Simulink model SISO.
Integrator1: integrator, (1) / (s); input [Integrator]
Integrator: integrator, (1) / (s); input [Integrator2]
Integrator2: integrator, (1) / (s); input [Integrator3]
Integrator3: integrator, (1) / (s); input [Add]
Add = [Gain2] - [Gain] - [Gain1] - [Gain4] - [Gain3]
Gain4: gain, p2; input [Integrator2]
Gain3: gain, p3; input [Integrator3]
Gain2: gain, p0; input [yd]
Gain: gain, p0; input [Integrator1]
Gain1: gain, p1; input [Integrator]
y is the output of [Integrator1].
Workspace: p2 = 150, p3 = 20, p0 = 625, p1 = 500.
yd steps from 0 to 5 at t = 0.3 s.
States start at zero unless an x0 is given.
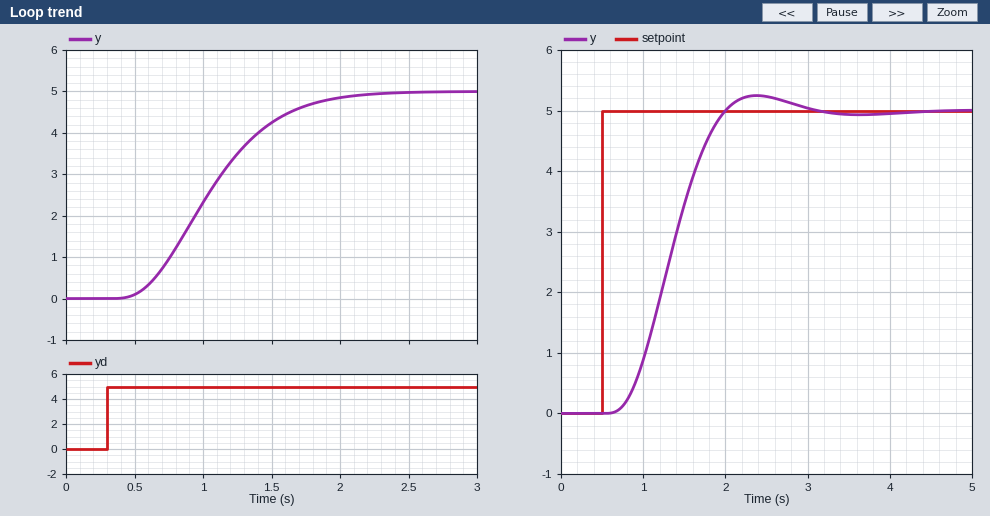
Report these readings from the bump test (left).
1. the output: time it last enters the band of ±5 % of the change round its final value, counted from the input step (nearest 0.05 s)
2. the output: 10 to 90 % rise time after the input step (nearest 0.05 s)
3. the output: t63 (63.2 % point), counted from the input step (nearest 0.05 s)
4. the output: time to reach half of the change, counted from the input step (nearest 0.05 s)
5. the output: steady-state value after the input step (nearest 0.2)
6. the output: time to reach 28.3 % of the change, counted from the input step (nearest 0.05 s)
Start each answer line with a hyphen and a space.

- 1.55 s
- 1.00 s
- 0.85 s
- 0.75 s
- 5.0
- 0.55 s
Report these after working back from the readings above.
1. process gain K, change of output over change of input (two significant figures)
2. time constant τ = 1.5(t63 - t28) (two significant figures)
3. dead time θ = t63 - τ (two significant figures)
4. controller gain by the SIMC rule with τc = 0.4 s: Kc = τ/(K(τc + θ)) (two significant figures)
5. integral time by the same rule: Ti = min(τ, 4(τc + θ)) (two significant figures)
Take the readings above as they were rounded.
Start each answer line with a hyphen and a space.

- 1.0
- 0.45 s
- 0.40 s
- 0.56
- 0.45 s
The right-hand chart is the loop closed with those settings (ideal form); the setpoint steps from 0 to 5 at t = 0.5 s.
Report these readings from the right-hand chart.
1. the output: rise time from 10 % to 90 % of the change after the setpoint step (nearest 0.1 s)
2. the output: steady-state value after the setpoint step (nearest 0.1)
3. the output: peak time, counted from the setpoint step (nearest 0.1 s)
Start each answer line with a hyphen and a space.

- 0.9 s
- 5.0
- 1.9 s
